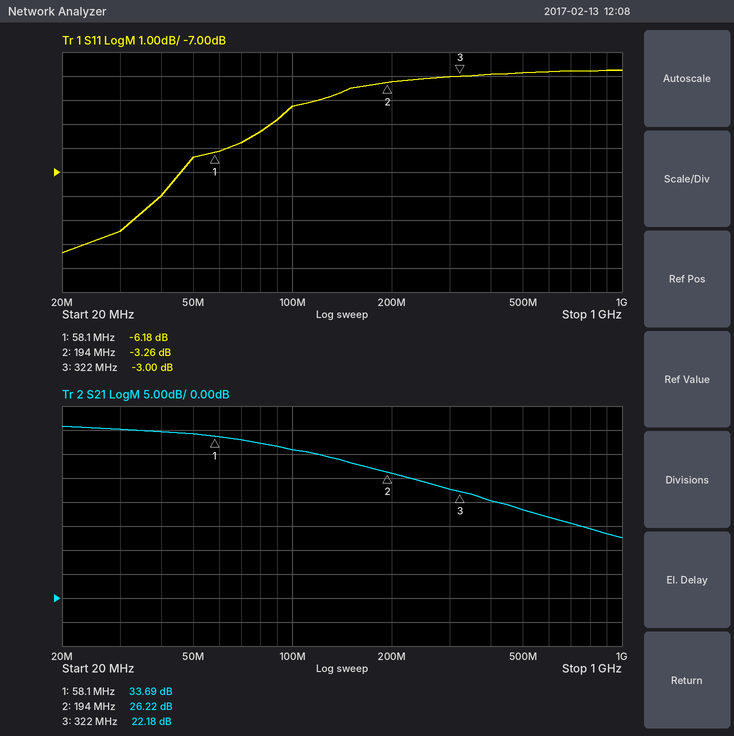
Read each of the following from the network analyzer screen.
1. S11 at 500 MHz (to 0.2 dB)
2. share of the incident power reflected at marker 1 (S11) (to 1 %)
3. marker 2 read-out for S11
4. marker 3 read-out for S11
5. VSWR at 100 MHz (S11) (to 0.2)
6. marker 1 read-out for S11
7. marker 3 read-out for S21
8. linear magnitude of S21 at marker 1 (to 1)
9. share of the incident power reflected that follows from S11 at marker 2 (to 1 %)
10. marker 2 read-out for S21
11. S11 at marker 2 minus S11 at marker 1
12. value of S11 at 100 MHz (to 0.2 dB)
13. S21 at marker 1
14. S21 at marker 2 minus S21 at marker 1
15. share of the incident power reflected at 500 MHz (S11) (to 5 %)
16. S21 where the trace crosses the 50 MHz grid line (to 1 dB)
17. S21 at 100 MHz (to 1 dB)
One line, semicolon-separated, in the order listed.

-2.8 dB; 24 %; -3.26 dB; -3.00 dB; 4.2; -6.18 dB; 22.18 dB; 48; 47 %; 26.22 dB; 2.92 dB; -4.2 dB; 33.69 dB; -7.47 dB; 50 %; 34 dB; 31 dB
